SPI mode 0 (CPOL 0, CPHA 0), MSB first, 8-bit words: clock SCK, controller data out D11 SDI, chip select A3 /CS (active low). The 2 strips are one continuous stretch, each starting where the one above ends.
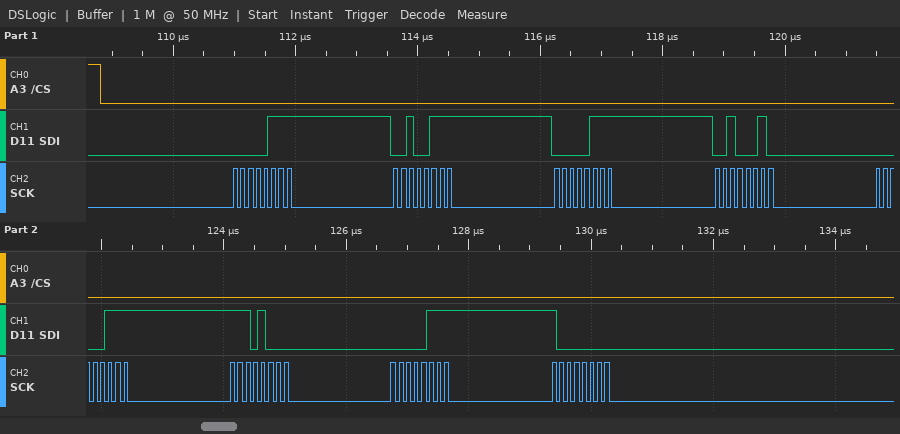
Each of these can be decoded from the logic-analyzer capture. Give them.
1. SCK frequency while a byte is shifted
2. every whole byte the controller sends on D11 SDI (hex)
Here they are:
8 MHz
07 27 07 22 07 E8 07 80
